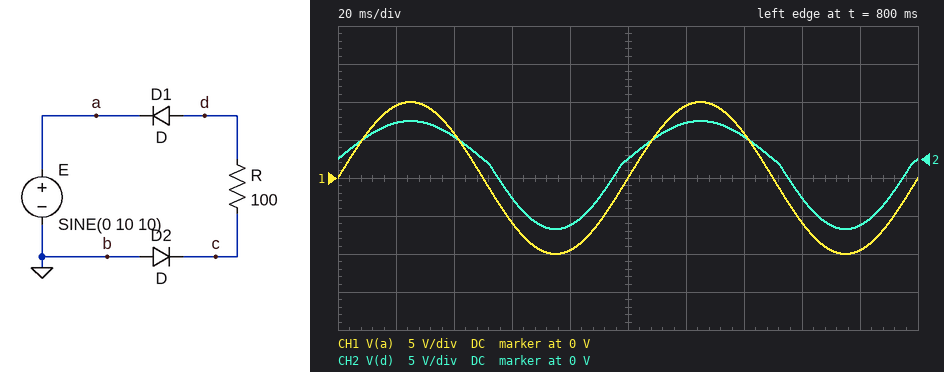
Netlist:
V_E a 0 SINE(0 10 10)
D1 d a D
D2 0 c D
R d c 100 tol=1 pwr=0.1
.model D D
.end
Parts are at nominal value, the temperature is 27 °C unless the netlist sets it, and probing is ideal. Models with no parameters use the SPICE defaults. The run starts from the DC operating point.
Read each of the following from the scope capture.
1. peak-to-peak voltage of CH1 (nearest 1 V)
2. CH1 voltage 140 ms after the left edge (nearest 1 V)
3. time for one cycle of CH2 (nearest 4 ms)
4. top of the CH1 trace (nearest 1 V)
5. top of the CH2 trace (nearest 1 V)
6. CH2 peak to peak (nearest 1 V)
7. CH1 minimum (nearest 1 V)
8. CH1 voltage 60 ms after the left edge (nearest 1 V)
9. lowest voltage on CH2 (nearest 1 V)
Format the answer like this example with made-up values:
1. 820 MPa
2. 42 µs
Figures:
1. 20 V
2. 6 V
3. 100 ms
4. 10 V
5. 5 V
6. 14 V
7. -10 V
8. -6 V
9. -9 V
